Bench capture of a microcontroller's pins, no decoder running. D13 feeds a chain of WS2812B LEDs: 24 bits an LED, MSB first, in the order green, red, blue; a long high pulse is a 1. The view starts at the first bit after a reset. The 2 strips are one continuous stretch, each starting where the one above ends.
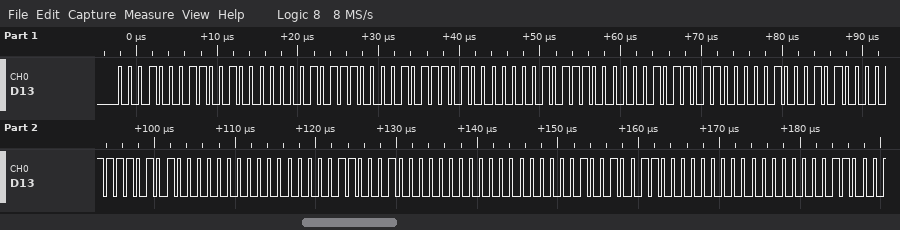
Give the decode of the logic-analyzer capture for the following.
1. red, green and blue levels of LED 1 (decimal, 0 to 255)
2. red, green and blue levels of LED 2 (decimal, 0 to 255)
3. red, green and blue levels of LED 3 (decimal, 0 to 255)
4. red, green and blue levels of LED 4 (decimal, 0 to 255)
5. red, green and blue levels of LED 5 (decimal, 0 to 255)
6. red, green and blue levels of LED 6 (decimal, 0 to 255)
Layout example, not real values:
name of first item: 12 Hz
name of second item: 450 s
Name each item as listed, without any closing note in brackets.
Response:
red, green and blue levels of LED 1: 144, 17, 23
red, green and blue levels of LED 2: 160, 11, 46
red, green and blue levels of LED 3: 176, 5, 69
red, green and blue levels of LED 4: 80, 15, 0
red, green and blue levels of LED 5: 64, 12, 0
red, green and blue levels of LED 6: 48, 9, 0
